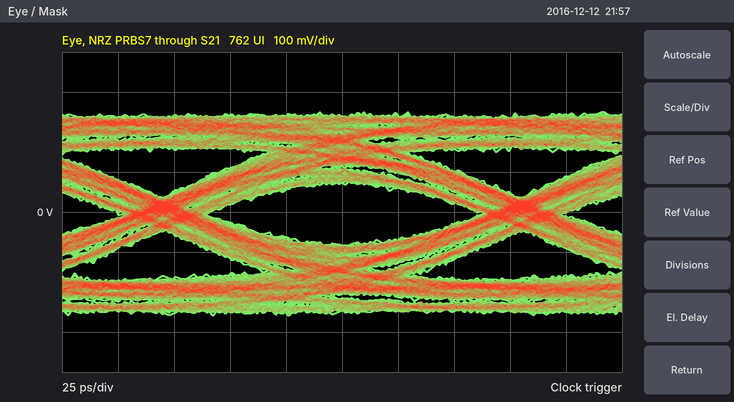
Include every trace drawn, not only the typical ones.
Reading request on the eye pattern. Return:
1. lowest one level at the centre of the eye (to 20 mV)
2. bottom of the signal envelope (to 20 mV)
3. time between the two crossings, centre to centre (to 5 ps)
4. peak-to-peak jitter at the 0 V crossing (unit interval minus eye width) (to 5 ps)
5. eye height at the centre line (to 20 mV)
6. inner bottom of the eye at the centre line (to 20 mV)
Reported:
80 mV
-260 mV
160 ps
40 ps
160 mV
-80 mV
